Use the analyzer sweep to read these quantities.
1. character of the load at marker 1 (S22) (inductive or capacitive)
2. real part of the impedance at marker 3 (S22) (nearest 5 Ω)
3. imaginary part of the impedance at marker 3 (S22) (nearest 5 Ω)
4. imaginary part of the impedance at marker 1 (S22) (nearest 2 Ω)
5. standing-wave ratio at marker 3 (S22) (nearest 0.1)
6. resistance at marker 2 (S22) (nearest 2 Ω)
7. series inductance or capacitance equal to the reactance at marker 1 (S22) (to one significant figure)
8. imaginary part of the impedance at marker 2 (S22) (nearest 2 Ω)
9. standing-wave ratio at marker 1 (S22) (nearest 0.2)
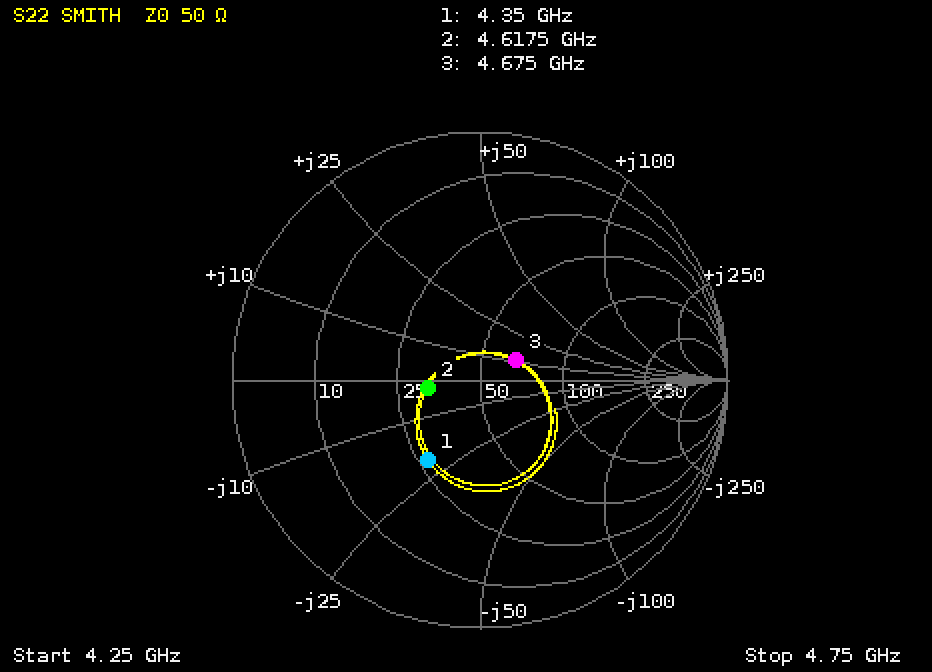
capacitive
65 Ω
+10 Ω
-20 Ω
1.4
32 Ω
2 pF
-2 Ω
2.2
